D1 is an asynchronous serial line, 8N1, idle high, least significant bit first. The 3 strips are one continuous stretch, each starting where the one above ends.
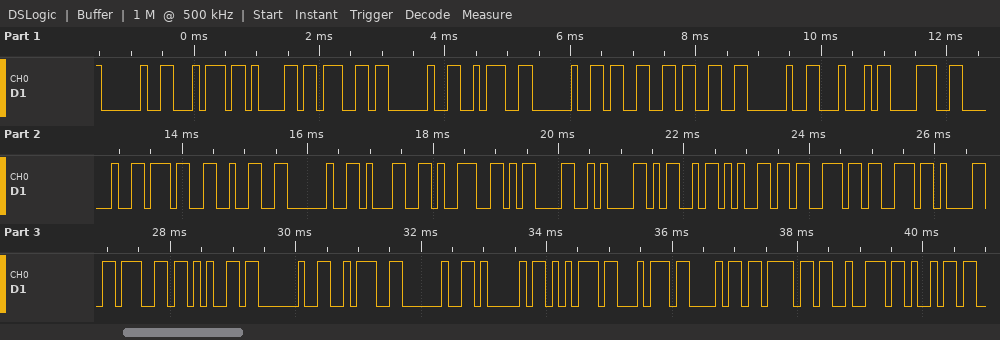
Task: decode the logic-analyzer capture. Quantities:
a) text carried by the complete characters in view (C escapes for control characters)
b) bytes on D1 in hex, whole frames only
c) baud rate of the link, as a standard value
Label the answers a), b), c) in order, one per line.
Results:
a) " tag : 33 D8 72 19\r\nMessage : Authori"
b) 20 74 61 67 20 3A 20 33 33 20 44 38 20 37 32 20 31 39 0D 0A 4D 65 73 73 61 67 65 20 3A 20 41 75 74 68 6F 72 69
c) 9600 baud
